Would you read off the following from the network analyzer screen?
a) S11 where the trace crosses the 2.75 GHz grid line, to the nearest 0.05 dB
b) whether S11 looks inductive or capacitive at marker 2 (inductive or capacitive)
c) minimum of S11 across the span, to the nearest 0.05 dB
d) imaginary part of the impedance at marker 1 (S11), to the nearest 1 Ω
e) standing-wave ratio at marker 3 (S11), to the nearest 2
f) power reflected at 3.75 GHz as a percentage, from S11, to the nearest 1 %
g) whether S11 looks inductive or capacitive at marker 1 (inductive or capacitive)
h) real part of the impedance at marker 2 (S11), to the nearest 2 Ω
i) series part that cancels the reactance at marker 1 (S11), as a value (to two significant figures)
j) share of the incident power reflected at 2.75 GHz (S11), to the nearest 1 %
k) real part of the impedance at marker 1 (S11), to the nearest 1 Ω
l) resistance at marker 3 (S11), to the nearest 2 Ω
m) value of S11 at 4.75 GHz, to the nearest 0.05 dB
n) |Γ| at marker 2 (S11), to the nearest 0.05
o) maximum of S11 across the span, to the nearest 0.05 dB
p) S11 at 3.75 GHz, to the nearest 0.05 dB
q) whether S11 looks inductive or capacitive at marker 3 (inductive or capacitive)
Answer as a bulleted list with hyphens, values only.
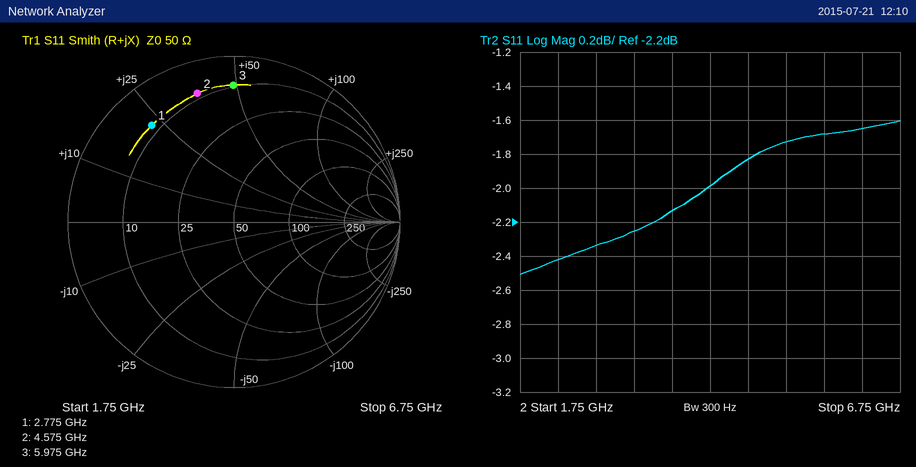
- -2.35 dB
- inductive
- -2.50 dB
- +23 Ω
- 10
- 61 %
- inductive
- 8 Ω
- 2.5 pF
- 58 %
- 8 Ω
- 10 Ω
- -1.85 dB
- 0.80
- -1.60 dB
- -2.15 dB
- inductive
